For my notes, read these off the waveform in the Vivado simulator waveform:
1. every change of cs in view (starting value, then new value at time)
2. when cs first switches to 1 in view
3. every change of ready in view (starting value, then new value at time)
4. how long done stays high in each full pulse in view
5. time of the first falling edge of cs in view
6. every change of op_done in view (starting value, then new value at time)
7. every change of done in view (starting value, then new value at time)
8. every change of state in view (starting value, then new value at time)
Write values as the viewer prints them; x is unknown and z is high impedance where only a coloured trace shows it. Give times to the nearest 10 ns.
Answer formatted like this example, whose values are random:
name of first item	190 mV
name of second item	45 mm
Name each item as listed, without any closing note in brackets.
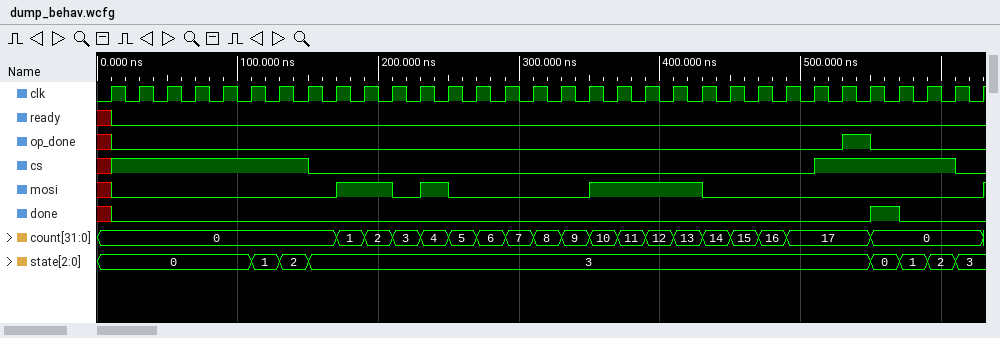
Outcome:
every change of cs in view	x, 1 at 10 ns, 0 at 150 ns, 1 at 510 ns, 0 at 610 ns
when cs first switches to 1 in view	10 ns
every change of ready in view	x, 0 at 10 ns
how long done stays high in each full pulse in view	20 ns
time of the first falling edge of cs in view	150 ns
every change of op_done in view	x, 0 at 10 ns, 1 at 530 ns, 0 at 550 ns
every change of done in view	x, 0 at 10 ns, 1 at 550 ns, 0 at 570 ns
every change of state in view	0, 1 at 110 ns, 2 at 130 ns, 3 at 150 ns, 0 at 550 ns, 1 at 570 ns, 2 at 590 ns, 3 at 610 ns
